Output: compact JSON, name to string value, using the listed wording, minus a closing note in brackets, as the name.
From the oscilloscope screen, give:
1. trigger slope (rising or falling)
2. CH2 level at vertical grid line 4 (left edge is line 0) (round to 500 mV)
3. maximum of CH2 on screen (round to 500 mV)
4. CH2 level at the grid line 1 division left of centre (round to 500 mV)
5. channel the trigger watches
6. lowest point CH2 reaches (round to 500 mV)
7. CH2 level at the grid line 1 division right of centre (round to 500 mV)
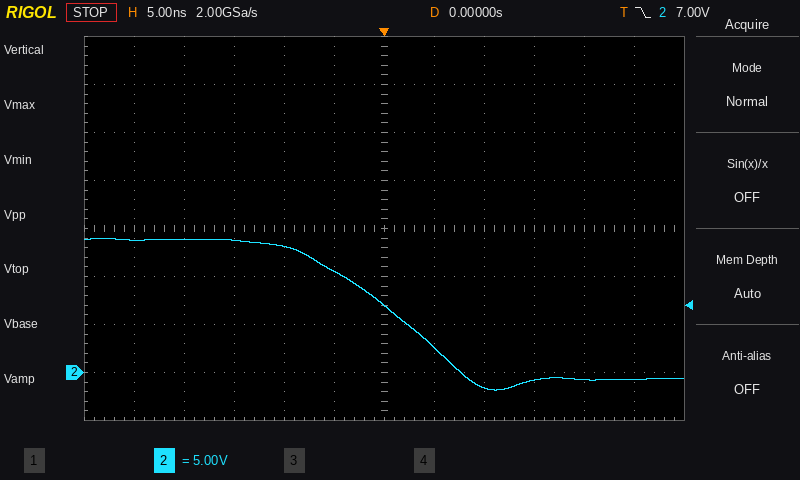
{"trigger slope": "falling", "CH2 level at vertical grid line 4 (left edge is line 0)": "13.0 V", "maximum of CH2 on screen": "14.0 V", "CH2 level at the grid line 1 division left of centre": "10.5 V", "channel the trigger watches": "CH2", "lowest point CH2 reaches": "-2.0 V", "CH2 level at the grid line 1 division right of centre": "2.5 V"}
